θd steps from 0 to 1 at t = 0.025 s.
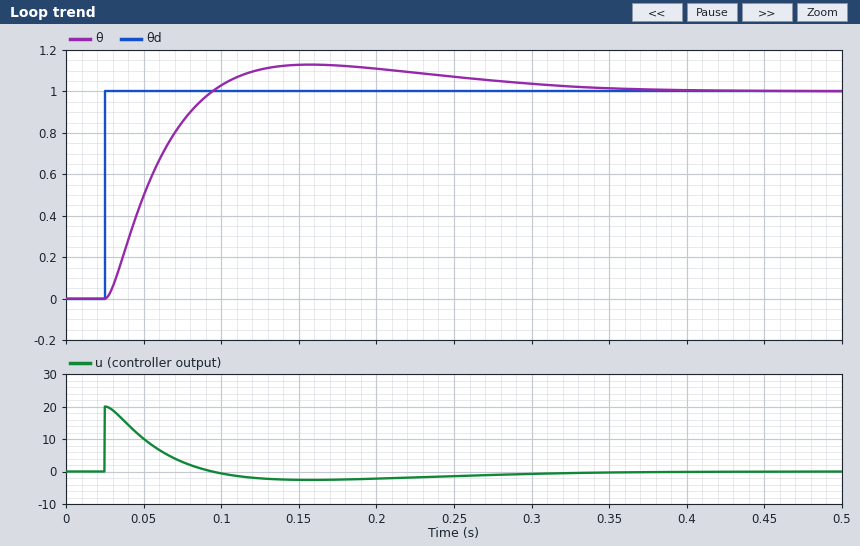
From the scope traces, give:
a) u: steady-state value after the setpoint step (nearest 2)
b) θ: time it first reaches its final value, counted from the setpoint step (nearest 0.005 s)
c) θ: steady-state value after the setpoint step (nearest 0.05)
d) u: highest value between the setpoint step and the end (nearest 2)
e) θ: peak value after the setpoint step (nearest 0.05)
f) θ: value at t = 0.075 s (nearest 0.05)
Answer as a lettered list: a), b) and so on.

a) 0
b) 0.070 s
c) 1.00
d) 20
e) 1.15
f) 0.85
